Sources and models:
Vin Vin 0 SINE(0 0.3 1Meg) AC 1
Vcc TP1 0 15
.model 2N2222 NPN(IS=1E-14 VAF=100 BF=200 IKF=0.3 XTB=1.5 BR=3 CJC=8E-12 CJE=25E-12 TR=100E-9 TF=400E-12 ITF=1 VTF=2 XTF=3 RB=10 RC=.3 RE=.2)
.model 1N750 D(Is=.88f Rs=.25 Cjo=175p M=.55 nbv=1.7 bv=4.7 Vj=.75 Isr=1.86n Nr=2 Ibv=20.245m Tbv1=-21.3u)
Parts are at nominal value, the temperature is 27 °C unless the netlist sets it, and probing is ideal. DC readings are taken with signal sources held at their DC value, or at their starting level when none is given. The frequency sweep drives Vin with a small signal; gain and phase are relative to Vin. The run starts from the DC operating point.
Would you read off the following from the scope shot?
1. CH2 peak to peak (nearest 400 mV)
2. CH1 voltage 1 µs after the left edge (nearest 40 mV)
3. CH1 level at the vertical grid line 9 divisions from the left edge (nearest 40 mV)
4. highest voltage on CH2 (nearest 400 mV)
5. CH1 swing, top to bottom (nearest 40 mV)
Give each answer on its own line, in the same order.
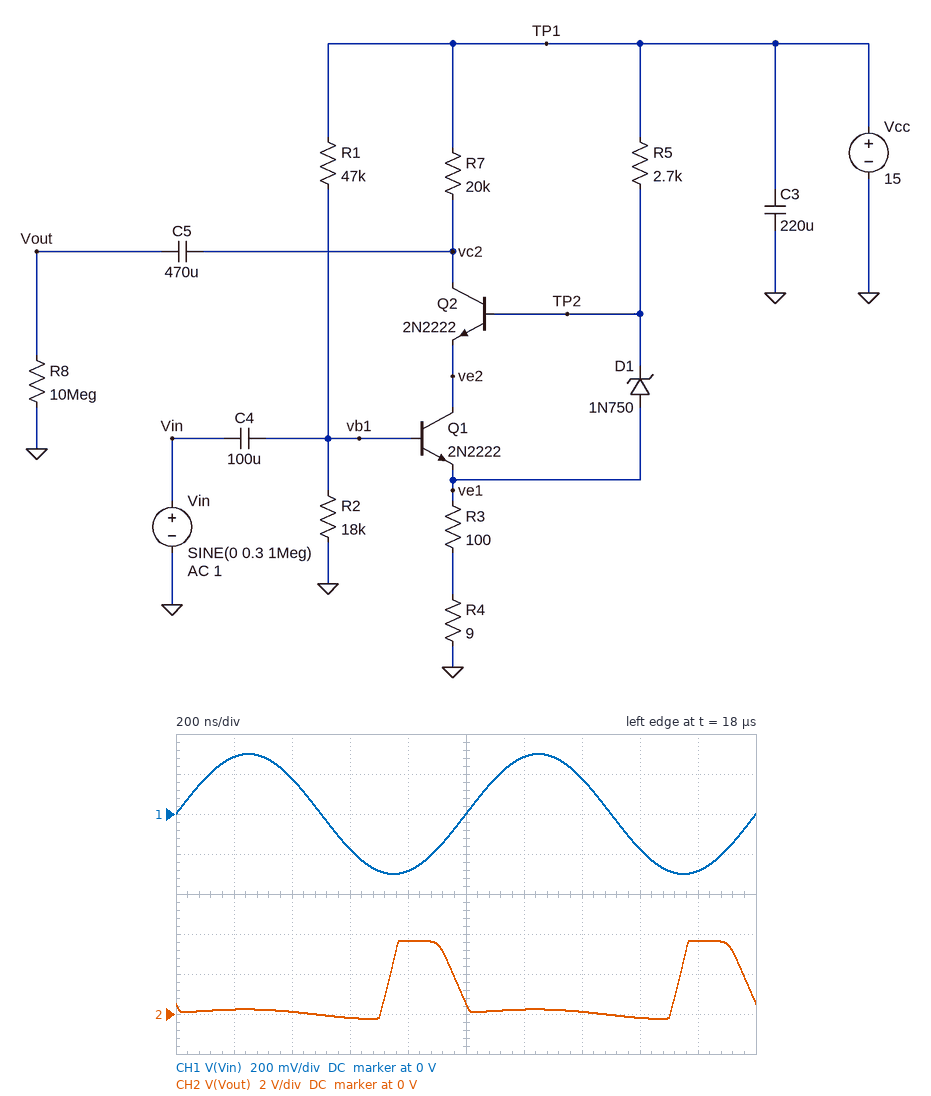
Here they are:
4.0 V
0 V
-280 mV
3.6 V
600 mV
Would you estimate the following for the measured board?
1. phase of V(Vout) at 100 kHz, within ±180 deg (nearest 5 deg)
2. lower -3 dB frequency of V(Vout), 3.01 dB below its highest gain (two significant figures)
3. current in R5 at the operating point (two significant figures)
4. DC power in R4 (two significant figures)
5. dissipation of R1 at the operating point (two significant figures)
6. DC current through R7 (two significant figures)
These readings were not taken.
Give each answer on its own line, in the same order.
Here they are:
115 deg
600 kHz
5.0 mA
320 µW
4.0 mW
710 µA
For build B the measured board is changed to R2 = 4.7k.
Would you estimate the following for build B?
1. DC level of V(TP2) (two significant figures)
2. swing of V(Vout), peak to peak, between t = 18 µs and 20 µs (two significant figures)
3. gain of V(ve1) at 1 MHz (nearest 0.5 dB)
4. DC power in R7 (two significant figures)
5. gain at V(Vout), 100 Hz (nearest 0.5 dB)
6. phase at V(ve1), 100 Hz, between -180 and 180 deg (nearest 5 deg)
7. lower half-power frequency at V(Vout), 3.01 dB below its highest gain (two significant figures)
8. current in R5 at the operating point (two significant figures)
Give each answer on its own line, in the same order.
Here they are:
3.0 V
3.9 V
-0.5 dB
8.1 mW
26.5 dB
0 deg
450 mHz
4.4 mA
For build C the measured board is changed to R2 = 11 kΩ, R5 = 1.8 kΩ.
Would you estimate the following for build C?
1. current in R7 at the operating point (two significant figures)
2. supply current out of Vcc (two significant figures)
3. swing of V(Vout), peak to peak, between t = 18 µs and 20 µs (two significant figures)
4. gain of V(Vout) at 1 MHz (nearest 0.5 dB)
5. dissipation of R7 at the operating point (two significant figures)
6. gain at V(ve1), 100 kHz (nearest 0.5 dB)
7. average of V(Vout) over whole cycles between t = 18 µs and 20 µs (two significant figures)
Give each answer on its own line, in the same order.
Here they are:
700 µA
8.3 mA
3.8 V
-0.5 dB
9.8 mW
-1.5 dB
820 mV
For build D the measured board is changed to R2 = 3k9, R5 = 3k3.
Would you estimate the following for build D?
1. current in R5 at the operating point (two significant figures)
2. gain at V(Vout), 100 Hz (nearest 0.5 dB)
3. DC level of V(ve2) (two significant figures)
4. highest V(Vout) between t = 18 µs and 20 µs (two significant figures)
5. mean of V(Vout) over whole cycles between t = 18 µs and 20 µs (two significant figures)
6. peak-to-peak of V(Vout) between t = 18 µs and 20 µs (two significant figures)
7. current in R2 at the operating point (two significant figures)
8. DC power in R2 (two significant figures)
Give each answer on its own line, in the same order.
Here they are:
3.1 mA
26.0 dB
4.1 V
270 mV
-1.7 V
3.9 V
280 µA
300 µW
